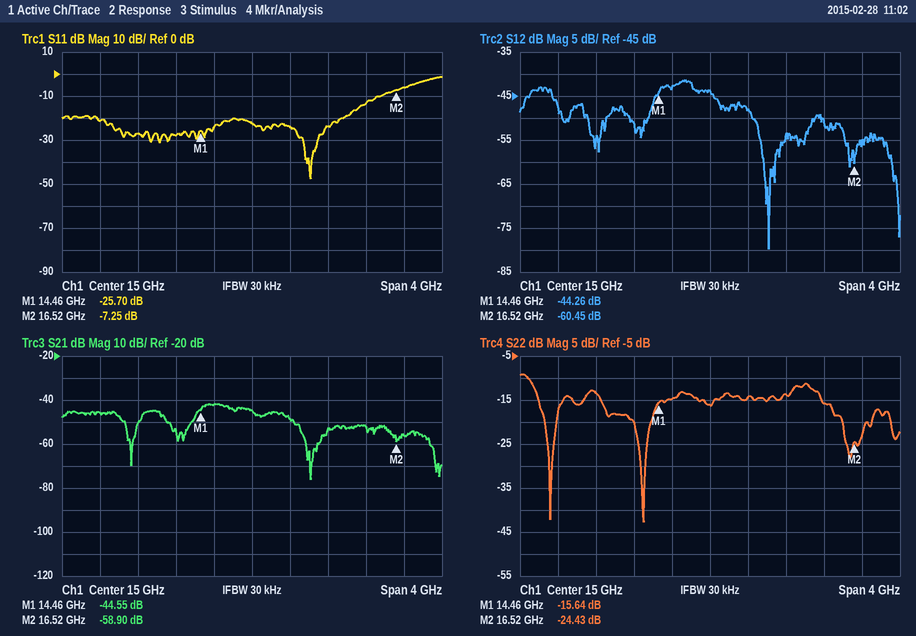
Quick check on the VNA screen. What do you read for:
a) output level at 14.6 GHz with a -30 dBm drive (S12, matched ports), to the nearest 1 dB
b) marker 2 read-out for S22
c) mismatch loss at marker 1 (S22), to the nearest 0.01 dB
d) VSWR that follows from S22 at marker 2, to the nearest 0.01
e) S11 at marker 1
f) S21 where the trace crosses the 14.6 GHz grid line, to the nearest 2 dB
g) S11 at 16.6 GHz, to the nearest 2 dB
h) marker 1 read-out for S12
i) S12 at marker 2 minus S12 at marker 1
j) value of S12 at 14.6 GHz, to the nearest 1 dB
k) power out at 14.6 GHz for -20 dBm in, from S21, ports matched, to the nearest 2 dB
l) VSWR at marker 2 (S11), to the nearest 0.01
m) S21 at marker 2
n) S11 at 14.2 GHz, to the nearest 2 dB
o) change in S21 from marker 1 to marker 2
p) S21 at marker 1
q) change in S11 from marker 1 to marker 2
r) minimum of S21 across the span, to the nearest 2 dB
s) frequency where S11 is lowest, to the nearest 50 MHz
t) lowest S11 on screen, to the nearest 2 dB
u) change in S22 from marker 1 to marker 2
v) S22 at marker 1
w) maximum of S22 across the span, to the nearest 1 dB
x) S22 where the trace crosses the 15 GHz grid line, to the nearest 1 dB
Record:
-73 dBm
-24.43 dB
0.12 dB
1.13
-25.70 dB
-42 dB
-6 dB
-44.26 dB
-16.19 dB
-43 dB
-62 dBm
2.53
-58.90 dB
-28 dB
-14.35 dB
-44.55 dB
18.45 dB
-76 dB
15.60 GHz
-48 dB
-8.79 dB
-15.64 dB
-9 dB
-16 dB
